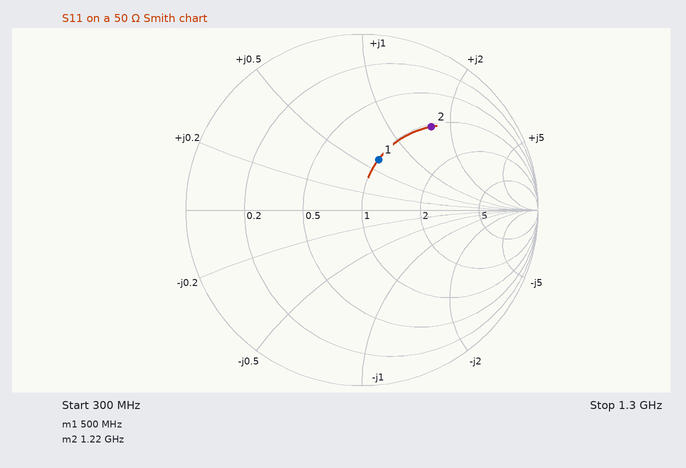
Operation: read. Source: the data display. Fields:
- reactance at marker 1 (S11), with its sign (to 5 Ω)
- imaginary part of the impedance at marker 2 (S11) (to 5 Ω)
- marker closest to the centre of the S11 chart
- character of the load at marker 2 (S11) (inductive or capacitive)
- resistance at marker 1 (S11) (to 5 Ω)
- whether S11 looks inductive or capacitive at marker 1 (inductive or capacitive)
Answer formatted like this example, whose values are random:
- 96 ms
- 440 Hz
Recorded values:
- +30 Ω
- +80 Ω
- marker 1
- inductive
- 50 Ω
- inductive
